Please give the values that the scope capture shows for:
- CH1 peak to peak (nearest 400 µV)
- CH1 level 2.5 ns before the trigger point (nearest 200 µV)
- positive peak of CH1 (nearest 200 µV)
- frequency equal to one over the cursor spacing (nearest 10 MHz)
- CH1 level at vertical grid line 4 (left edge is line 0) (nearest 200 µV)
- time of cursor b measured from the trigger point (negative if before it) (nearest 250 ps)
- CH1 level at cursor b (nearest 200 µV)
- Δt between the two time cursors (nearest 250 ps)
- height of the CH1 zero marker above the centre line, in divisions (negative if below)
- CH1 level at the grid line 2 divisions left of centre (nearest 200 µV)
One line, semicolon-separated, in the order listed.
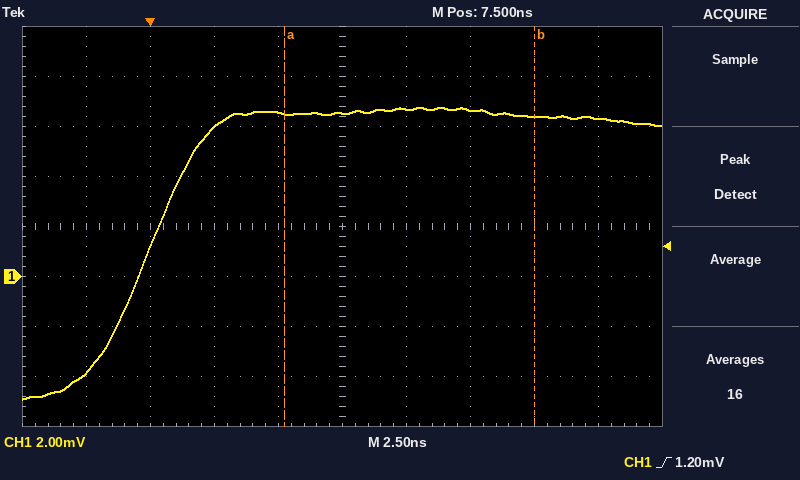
11.6 mV; -3.8 mV; 6.8 mV; 100 MHz; 6.6 mV; +15.00 ns; 6.4 mV; 9.75 ns; -1.0 div; 6.0 mV
